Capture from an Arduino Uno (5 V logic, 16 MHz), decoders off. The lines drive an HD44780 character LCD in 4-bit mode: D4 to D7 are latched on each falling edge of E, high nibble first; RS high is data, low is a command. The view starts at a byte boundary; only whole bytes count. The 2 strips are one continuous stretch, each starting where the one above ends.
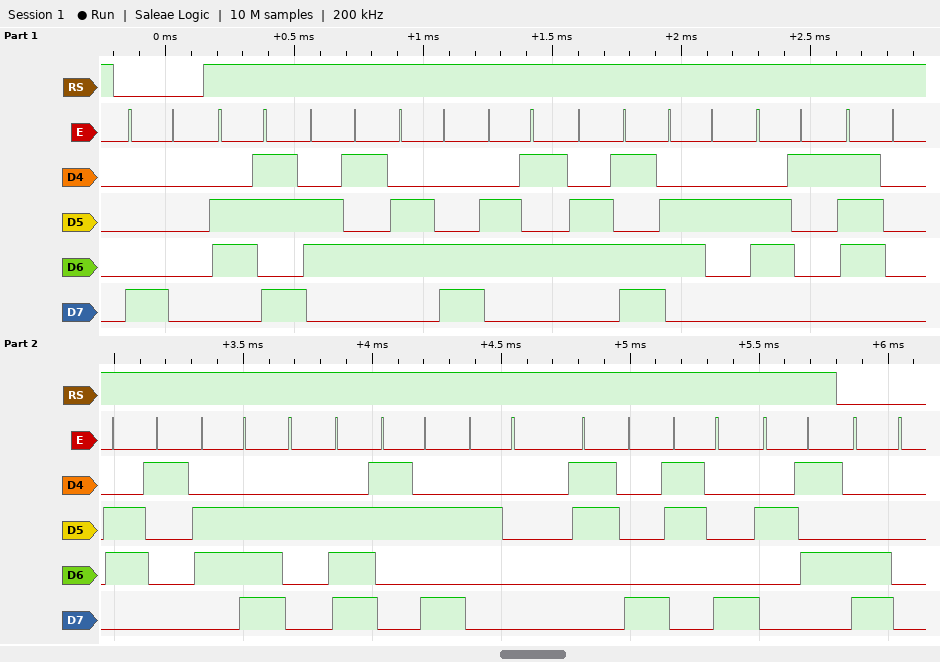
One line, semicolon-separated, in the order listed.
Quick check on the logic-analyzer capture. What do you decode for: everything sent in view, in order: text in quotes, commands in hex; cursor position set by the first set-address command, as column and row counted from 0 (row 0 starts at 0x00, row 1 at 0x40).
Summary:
0x80 "kelembapan.: 88%" 0xC0; column 0, row 0
